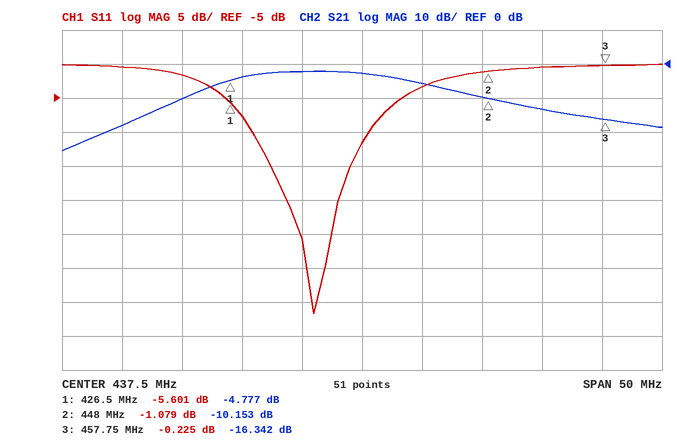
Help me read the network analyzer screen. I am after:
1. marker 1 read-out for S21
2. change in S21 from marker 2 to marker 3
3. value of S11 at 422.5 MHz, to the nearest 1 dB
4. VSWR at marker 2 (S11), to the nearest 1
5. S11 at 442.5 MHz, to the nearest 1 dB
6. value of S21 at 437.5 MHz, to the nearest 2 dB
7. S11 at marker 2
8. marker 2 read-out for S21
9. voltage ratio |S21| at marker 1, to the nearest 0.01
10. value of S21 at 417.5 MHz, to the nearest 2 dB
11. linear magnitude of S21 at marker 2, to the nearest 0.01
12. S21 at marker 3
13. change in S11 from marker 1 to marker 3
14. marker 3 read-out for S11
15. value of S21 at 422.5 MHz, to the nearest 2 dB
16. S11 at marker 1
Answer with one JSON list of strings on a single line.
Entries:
["-4.777 dB", "-6.189 dB", "-2 dB", "16", "-3 dB", "-2 dB", "-1.079 dB", "-10.153 dB", "0.58", "-18 dB", "0.31", "-16.342 dB", "5.376 dB", "-0.225 dB", "-10 dB", "-5.601 dB"]
